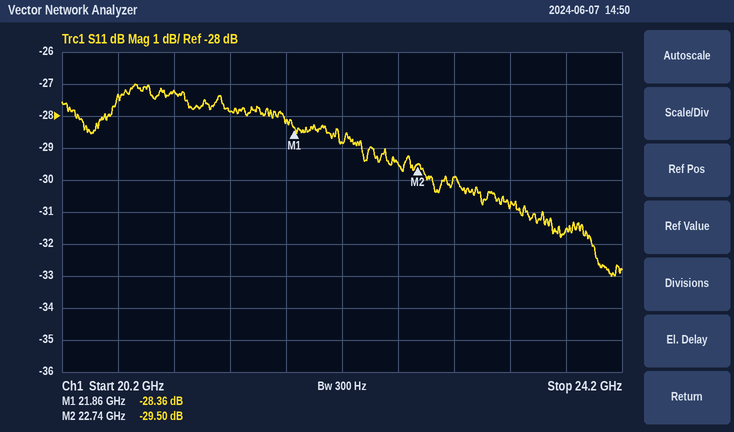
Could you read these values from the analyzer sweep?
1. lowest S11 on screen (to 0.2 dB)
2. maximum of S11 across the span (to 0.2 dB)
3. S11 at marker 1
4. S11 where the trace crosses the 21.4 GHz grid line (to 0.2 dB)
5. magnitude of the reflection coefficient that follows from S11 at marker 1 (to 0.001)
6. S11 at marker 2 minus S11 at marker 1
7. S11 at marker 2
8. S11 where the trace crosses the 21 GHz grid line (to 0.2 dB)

-33.0 dB
-27.0 dB
-28.36 dB
-27.8 dB
0.038
-1.14 dB
-29.50 dB
-27.2 dB
